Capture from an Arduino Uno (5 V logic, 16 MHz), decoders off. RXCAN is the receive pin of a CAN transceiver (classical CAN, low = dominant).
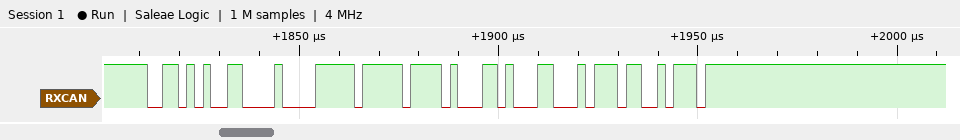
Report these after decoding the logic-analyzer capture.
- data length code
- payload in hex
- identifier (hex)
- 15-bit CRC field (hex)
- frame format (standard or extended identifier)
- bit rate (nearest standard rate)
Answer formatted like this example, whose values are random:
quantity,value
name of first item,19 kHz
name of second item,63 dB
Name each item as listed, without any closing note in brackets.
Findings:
quantity,value
data length code,4
payload in hex,3F FF 46 8C
identifier,0x353
15-bit CRC field,0x2ECB
frame format,standard
bit rate,500 kbit/s
